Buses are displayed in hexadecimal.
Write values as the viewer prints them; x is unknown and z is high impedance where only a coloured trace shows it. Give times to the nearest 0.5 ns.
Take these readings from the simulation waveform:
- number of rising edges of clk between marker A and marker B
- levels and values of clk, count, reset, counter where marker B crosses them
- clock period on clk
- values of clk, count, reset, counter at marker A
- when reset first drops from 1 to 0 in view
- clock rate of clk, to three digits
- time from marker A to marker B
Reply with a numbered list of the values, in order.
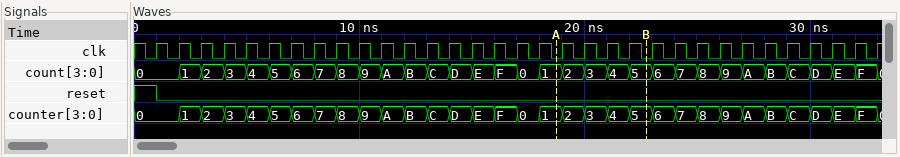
1. 4
2. clk=0, count=5, reset=0, counter=5
3. 1 ns
4. clk=0, count=1, reset=0, counter=1
5. 1 ns
6. 1.00 GHz
7. 4 ns
